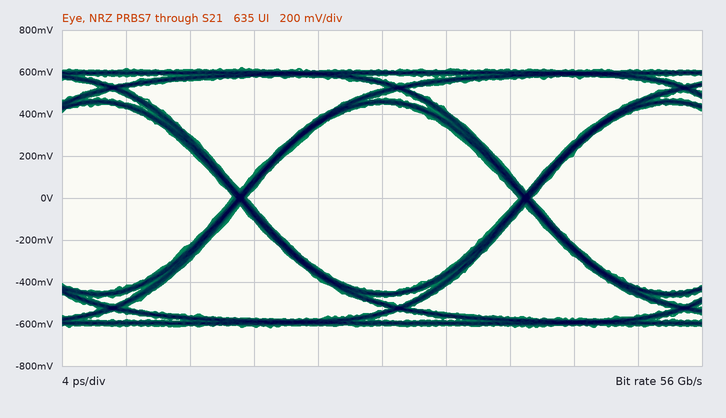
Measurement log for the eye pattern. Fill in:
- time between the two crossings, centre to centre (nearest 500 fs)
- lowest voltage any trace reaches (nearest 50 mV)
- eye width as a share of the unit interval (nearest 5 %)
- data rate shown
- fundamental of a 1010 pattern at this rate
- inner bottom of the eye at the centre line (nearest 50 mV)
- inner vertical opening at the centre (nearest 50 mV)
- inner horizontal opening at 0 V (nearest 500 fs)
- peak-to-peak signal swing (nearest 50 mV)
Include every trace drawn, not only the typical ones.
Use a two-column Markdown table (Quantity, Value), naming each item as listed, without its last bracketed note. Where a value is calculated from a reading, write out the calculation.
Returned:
| Quantity | Value |
|---|---|
| time between the two crossings, centre to centre | 18.0 ps |
| lowest voltage any trace reaches | -600 mV |
| eye width as a share of the unit interval | 17.0 ps / 18.0 ps ≈ 94.4 %, so 95 % to the nearest 5 % |
| data rate shown | 56 Gb/s |
| fundamental of a 1010 pattern at this rate | 28 GHz |
| inner bottom of the eye at the centre line | -450 mV |
| inner vertical opening at the centre | 900 mV |
| inner horizontal opening at 0 V | 17.0 ps |
| peak-to-peak signal swing | 1.25 V |
